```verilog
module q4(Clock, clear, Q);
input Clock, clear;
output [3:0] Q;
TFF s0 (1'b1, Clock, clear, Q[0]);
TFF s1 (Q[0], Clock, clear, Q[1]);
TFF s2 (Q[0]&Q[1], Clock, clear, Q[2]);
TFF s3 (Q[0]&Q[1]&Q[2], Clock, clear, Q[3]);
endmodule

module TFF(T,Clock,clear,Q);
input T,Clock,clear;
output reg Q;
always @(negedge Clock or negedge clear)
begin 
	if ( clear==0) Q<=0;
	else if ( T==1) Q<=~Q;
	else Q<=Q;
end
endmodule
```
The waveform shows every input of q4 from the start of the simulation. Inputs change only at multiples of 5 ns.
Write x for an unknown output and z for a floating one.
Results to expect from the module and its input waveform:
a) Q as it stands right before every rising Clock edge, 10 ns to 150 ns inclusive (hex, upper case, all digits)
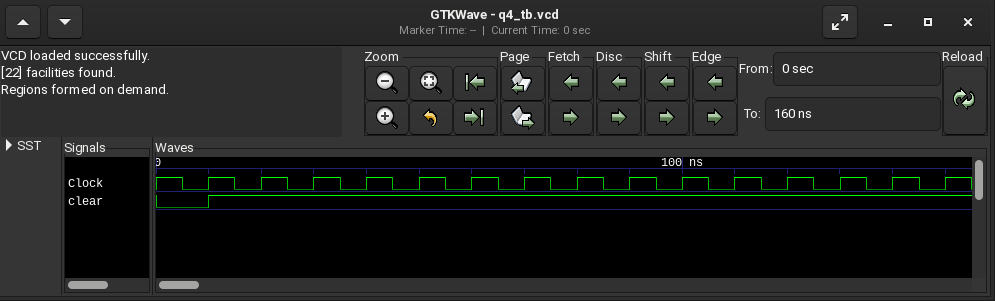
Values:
0, 1, 2, 3, 4, 5, 6, 7, 8, 9, A, B, C, D, E
